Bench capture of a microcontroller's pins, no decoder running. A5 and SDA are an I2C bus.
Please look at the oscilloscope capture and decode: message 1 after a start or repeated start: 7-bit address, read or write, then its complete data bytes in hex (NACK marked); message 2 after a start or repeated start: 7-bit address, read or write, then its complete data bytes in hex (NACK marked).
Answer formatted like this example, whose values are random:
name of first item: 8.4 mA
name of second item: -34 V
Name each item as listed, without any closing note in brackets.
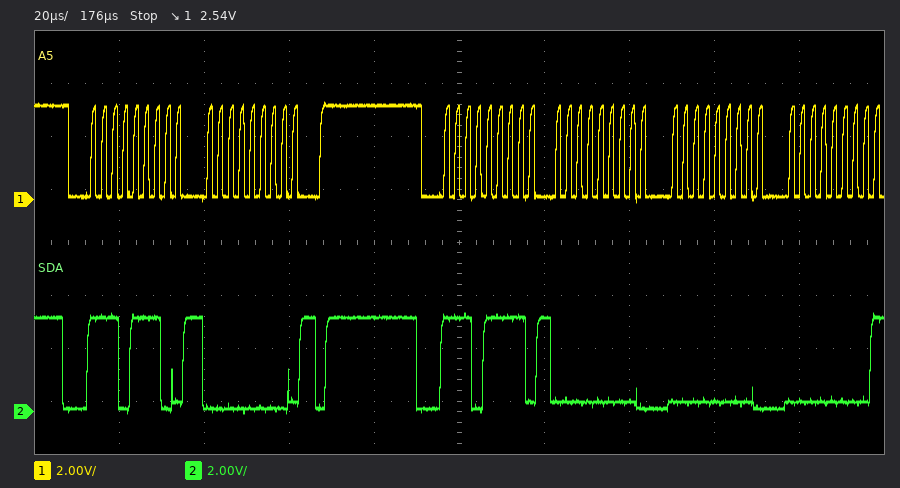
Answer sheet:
message 1 after a start or repeated start: 7-bit address, read or write, then its complete data bytes in hex: 0x77 write: 00
message 2 after a start or repeated start: 7-bit address, read or write, then its complete data bytes in hex: 0x77 read: 00 00 00 NACK
